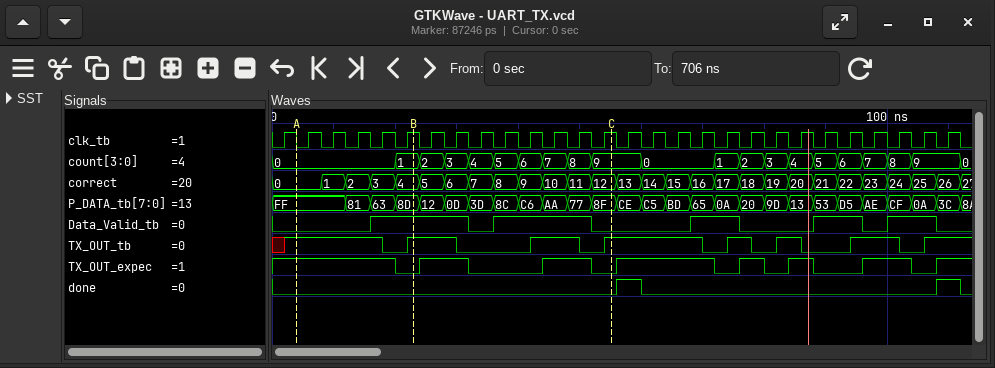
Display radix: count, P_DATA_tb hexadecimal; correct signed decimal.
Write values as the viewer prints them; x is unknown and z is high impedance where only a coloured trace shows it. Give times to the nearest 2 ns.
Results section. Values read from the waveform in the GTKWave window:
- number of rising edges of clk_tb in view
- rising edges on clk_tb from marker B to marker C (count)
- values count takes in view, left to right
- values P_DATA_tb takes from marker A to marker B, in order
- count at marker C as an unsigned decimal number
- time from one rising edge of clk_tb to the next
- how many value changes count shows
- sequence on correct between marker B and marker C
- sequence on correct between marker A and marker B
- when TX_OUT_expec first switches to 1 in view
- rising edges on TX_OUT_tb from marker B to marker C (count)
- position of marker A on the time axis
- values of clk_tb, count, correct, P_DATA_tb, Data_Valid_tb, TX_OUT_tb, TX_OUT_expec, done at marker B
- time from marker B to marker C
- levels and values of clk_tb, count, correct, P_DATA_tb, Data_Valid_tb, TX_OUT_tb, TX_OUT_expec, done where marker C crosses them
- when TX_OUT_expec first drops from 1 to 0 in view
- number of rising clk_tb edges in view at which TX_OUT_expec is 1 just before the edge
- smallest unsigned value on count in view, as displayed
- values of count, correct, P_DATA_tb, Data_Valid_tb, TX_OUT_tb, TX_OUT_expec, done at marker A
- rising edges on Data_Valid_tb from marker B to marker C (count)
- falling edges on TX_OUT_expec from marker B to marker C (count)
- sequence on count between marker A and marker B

28
8
0, 1, 2, 3, 4, 5, 6, 7, 8, 9, 0, 1, 2, 3, 4, 5, 6, 7, 8, 9, 0
FF, 81, 63, 8D
9
4 ns
20
4, 5, 6, 7, 8, 9, 10, 11, 12
0, 1, 2, 3, 4
24 ns
2
4 ns
clk_tb=1, count=1, correct=4, P_DATA_tb=8D, Data_Valid_tb=1, TX_OUT_tb=1, TX_OUT_expec=0, done=0
32 ns
clk_tb=1, count=9, correct=12, P_DATA_tb=8F, Data_Valid_tb=0, TX_OUT_tb=1, TX_OUT_expec=0, done=0
20 ns
18
0
count=0, correct=0, P_DATA_tb=FF, Data_Valid_tb=0, TX_OUT_tb=1, TX_OUT_expec=1, done=0
1
2
0, 1
